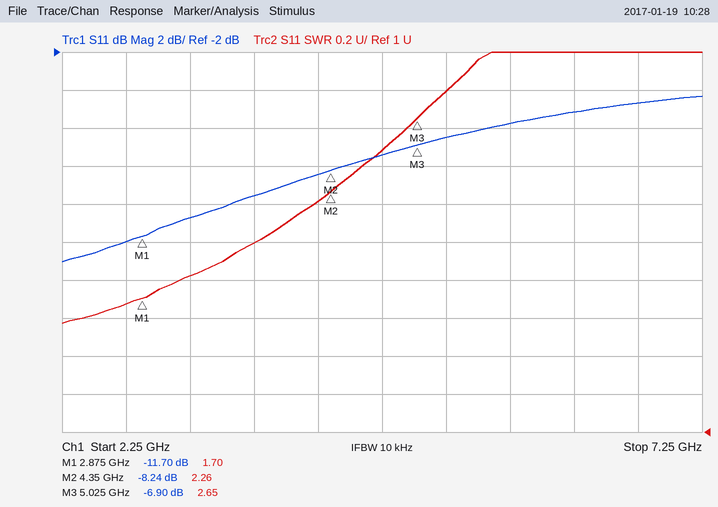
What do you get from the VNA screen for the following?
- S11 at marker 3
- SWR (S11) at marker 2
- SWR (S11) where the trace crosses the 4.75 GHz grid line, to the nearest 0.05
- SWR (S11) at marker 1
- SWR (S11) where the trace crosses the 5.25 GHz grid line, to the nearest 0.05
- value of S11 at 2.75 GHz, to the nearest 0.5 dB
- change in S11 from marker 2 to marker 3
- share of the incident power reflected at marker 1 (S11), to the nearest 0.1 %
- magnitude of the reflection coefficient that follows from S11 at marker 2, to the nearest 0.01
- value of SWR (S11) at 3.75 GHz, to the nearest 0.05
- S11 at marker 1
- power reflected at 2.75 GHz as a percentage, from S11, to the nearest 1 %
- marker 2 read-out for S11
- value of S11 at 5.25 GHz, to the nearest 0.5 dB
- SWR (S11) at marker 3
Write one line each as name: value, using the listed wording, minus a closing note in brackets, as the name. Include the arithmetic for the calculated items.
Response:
S11 at marker 3: -6.90 dB
SWR (S11) at marker 2: 2.26
SWR (S11) where the trace crosses the 4.75 GHz grid line, to the nearest 0.05: 2.50
SWR (S11) at marker 1: 1.70
SWR (S11) where the trace crosses the 5.25 GHz grid line, to the nearest 0.05: 2.80
value of S11 at 2.75 GHz, to the nearest 0.5 dB: -12.0 dB
change in S11 from marker 2 to marker 3: -6.9 − (-8.24) = 1.34 dB
share of the incident power reflected at marker 1 (S11), to the nearest 0.1 %: 10^(-11.7/10) ≈ 6.8 %
magnitude of the reflection coefficient that follows from S11 at marker 2, to the nearest 0.01: 10^(-8.24/20) ≈ 0.39
value of SWR (S11) at 3.75 GHz, to the nearest 0.05: 2.00
S11 at marker 1: -11.70 dB
power reflected at 2.75 GHz as a percentage, from S11, to the nearest 1 %: 10^(-12/10) ≈ 6 %
marker 2 read-out for S11: -8.24 dB
value of S11 at 5.25 GHz, to the nearest 0.5 dB: -6.5 dB
SWR (S11) at marker 3: 2.65
